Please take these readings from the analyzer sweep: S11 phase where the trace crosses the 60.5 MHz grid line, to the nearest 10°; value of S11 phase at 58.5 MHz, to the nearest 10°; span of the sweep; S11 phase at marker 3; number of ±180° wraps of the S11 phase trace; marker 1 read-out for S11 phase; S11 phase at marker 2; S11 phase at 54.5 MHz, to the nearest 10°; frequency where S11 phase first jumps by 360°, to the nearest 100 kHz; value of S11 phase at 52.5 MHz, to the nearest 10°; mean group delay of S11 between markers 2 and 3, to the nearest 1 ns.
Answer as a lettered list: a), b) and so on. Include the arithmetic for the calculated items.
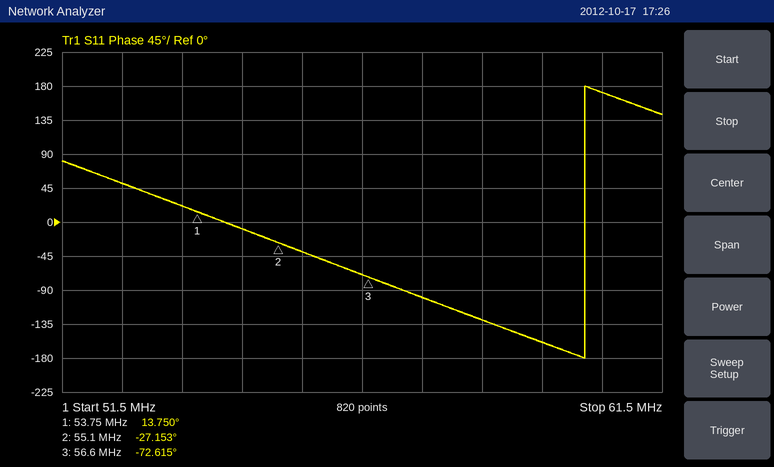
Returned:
a) 170°
b) -130°
c) 10 MHz
d) -72.615°
e) 1
f) 13.750°
g) -27.153°
h) -10°
i) 60.2 MHz
j) 50°
k) −(-72.615° − (-27.153°))/(360° × 1.5 MHz) ≈ 84 ns
